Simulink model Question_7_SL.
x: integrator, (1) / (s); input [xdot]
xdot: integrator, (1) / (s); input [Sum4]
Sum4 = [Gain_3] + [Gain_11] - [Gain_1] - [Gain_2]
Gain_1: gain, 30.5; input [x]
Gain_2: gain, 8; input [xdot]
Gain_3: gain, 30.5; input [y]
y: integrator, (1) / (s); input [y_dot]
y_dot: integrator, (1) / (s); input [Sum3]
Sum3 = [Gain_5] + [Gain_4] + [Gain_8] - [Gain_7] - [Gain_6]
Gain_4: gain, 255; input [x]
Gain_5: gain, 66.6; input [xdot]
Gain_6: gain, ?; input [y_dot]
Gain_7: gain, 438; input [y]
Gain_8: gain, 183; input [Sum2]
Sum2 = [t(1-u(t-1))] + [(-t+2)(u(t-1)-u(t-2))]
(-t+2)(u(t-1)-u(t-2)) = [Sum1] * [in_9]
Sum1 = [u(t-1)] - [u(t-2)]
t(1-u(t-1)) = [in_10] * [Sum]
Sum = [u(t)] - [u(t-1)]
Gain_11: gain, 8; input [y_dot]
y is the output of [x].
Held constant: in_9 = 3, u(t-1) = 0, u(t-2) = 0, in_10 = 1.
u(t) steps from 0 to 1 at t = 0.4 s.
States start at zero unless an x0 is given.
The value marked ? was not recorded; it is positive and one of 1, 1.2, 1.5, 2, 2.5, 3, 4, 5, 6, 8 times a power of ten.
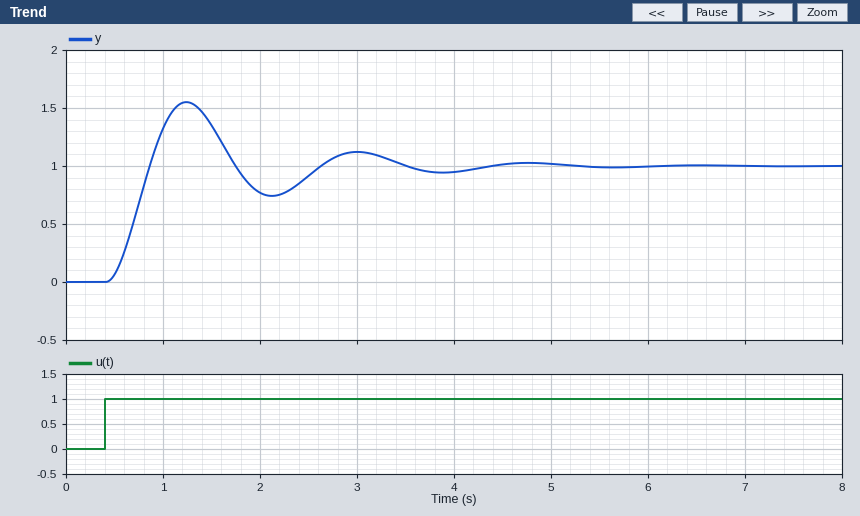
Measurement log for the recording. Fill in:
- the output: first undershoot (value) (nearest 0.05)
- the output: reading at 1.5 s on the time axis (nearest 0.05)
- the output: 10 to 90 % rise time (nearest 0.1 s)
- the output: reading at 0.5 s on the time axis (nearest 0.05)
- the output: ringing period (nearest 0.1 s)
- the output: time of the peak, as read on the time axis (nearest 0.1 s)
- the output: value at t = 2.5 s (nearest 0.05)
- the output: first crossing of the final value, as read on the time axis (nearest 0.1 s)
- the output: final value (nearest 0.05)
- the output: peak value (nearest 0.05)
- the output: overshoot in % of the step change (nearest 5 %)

0.75
1.35
0.3 s
0.05
1.8 s
1.2 s
0.90
0.9 s
1.00
1.55
55 %
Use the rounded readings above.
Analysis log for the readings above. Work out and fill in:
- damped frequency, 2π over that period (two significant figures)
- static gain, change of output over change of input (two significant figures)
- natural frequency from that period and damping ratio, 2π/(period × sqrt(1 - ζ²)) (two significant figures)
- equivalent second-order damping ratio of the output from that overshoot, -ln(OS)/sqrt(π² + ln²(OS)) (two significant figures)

3.5 rad/s
1.0
3.6 rad/s
0.19
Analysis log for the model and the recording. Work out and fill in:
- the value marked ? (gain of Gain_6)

80
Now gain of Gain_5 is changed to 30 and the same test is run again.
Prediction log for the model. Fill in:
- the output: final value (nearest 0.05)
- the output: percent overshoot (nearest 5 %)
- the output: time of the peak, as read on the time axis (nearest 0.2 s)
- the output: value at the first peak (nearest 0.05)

1.00
15 %
1.4 s
1.15
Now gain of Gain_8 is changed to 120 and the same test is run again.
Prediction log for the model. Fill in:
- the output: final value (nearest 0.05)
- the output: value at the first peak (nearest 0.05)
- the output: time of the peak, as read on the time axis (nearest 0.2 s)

0.65
1.00
1.2 s
